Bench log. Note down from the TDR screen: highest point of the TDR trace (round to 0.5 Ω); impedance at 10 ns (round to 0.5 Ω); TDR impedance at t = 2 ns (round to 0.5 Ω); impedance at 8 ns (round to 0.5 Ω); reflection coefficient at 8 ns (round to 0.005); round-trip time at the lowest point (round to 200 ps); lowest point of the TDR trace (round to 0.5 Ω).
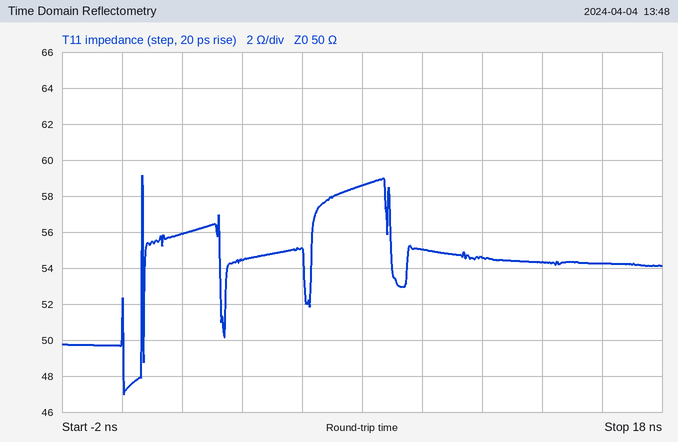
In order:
59.0 Ω
55.0 Ω
56.0 Ω
58.5 Ω
+0.080
0.0 ns
47.0 Ω
